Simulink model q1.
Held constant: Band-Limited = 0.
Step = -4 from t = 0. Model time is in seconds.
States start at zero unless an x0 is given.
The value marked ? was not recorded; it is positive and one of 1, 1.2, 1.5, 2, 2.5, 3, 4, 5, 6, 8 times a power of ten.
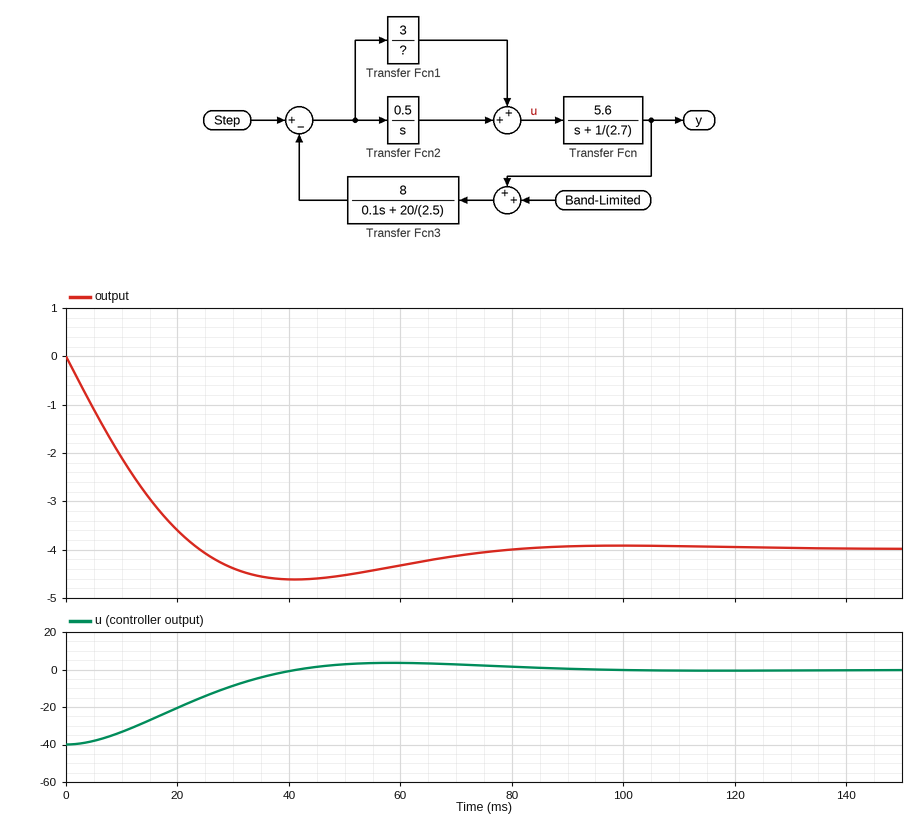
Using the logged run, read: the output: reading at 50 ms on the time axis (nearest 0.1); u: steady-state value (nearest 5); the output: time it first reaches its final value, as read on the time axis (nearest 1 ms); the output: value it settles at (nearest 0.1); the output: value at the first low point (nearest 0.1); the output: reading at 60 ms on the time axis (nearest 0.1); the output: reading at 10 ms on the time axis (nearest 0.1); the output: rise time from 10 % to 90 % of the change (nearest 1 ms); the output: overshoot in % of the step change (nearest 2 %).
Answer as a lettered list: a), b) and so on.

a) -4.5
b) 0
c) 24 ms
d) -4.0
e) -4.6
f) -4.3
g) -2.1
h) 18 ms
i) 16 %
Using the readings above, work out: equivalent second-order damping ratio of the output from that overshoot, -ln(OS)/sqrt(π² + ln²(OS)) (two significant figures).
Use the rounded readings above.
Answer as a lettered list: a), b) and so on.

a) 0.50
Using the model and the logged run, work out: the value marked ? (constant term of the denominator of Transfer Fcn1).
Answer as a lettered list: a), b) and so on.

a) 0.3
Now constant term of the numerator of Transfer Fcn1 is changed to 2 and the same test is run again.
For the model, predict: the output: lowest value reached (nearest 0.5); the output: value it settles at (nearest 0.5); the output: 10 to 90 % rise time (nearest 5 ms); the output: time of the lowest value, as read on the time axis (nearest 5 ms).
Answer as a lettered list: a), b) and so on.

a) -4.0
b) -4.0
c) 30 ms
d) 65 ms
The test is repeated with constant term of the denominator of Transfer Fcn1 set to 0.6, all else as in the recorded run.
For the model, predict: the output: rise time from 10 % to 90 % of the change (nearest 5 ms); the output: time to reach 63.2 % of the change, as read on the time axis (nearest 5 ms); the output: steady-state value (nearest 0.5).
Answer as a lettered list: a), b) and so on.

a) 45 ms
b) 25 ms
c) -4.0
